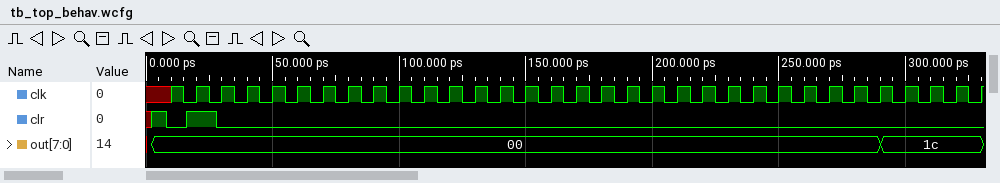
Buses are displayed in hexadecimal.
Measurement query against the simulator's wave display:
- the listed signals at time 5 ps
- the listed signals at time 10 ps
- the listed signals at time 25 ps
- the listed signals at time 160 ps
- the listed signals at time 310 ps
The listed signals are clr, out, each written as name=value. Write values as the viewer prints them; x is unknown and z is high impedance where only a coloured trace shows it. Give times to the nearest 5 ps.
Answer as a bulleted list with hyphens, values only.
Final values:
- clr=1, out=00
- clr=0, out=00
- clr=1, out=00
- clr=0, out=00
- clr=0, out=1c
